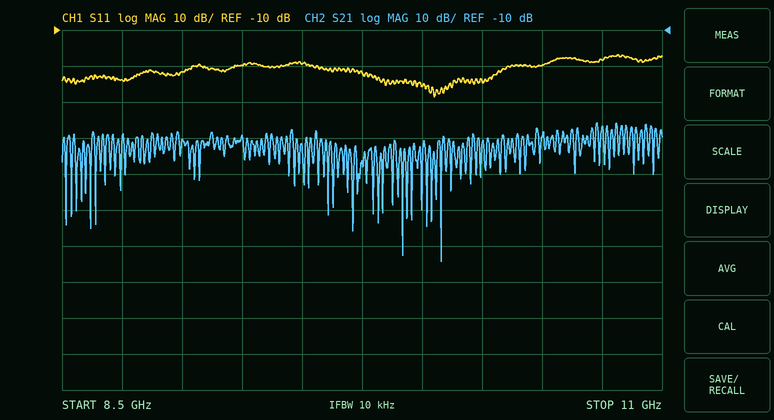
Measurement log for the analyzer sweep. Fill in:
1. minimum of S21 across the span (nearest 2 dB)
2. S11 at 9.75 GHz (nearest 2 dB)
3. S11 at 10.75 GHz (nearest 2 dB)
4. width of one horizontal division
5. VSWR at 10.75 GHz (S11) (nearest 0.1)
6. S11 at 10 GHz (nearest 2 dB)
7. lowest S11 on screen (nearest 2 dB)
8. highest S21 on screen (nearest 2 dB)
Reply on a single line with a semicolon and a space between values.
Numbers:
-74 dB; -22 dB; -18 dB; 250 MHz; 1.3; -26 dB; -28 dB; -36 dB
